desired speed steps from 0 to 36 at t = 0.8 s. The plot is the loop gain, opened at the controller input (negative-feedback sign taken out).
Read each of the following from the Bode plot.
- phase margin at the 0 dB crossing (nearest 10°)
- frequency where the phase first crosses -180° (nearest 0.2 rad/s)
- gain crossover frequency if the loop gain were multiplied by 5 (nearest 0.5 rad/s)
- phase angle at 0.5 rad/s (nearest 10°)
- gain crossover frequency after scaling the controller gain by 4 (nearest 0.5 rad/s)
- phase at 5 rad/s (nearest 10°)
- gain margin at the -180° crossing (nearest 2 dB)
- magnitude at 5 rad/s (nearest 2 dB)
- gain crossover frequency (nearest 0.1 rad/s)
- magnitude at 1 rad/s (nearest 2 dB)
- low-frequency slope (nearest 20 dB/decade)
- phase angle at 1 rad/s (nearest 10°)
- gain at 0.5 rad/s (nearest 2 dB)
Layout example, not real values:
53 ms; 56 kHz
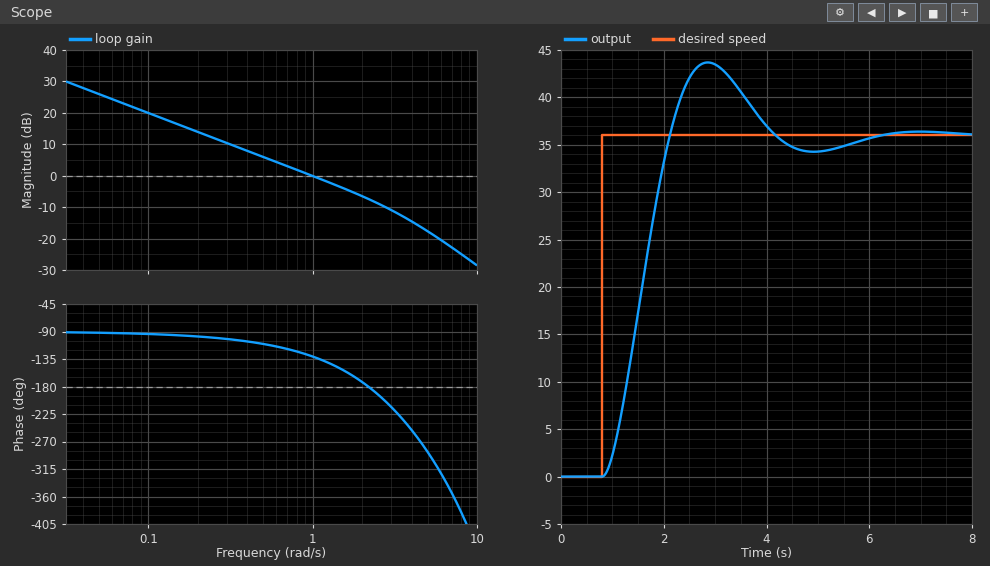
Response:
50°; 2.2 rad/s; 4.0 rad/s; -110°; 3.5 rad/s; -290°; 8 dB; -18 dB; 1.0 rad/s; 0 dB; -20 dB/decade; -130°; 6 dB
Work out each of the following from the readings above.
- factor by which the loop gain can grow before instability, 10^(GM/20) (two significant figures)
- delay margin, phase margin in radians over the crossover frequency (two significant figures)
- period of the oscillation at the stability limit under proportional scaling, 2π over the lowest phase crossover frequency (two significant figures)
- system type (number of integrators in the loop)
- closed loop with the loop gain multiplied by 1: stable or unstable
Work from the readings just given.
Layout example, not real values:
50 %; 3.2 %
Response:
2.5; 0.87 s; 2.9 s; 1; stable
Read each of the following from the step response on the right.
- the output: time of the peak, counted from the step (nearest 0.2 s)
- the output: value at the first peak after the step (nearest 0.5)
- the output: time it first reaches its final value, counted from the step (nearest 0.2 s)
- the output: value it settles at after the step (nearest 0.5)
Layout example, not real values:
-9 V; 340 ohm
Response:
2.0 s; 43.5; 1.4 s; 36.0
